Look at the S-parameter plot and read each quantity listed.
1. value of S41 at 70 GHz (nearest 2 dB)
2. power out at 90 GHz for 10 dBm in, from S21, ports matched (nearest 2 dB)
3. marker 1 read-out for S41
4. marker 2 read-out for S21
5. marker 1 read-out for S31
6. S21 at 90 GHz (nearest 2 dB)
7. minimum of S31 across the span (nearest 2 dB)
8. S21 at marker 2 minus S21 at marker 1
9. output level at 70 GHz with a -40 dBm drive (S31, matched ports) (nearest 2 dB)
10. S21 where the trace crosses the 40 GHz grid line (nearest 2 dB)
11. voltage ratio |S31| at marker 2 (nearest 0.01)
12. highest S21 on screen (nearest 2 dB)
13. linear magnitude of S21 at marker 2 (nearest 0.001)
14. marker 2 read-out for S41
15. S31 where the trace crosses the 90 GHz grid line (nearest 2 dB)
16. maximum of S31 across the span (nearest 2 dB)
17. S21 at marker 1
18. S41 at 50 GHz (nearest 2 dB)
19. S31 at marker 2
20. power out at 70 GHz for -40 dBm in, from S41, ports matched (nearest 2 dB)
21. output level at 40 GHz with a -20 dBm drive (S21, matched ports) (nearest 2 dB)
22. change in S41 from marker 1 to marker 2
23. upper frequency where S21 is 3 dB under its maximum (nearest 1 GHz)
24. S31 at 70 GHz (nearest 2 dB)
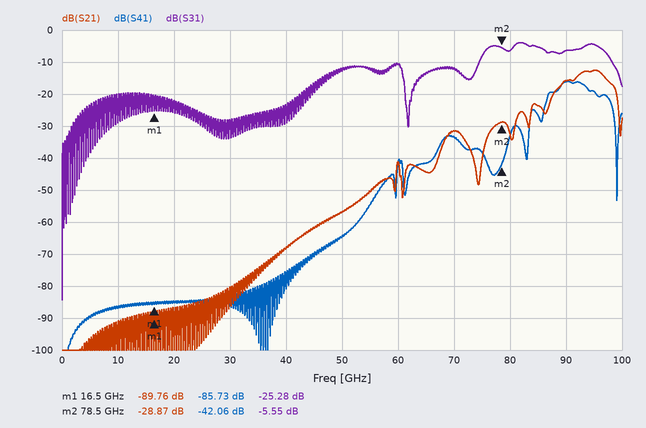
-34 dB
-6 dBm
-85.73 dB
-28.87 dB
-25.28 dB
-16 dB
-84 dB
60.89 dB
-52 dBm
-68 dB
0.53
-12 dB
0.036
-42.06 dB
-6 dB
-4 dB
-89.76 dB
-64 dB
-5.55 dB
-74 dBm
-88 dBm
43.67 dB
97 GHz
-12 dB
